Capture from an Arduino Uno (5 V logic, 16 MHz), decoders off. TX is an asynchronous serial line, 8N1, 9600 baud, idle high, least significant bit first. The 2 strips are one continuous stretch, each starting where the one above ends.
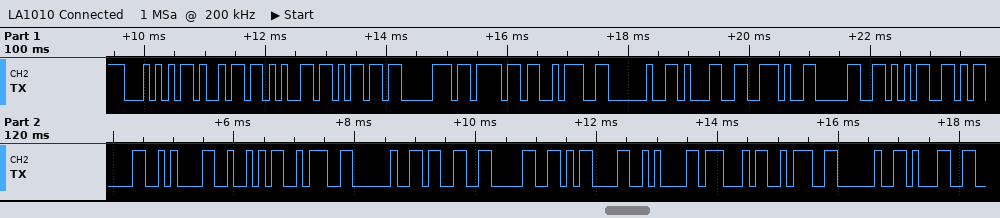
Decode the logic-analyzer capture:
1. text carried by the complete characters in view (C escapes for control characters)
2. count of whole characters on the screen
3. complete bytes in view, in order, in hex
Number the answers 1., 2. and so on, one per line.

1. "Tiempo: 1.05\r\nR: 30\r\nG: 1"
2. 25
3. 54 69 65 6D 70 6F 3A 20 31 2E 30 35 0D 0A 52 3A 20 33 30 0D 0A 47 3A 20 31
